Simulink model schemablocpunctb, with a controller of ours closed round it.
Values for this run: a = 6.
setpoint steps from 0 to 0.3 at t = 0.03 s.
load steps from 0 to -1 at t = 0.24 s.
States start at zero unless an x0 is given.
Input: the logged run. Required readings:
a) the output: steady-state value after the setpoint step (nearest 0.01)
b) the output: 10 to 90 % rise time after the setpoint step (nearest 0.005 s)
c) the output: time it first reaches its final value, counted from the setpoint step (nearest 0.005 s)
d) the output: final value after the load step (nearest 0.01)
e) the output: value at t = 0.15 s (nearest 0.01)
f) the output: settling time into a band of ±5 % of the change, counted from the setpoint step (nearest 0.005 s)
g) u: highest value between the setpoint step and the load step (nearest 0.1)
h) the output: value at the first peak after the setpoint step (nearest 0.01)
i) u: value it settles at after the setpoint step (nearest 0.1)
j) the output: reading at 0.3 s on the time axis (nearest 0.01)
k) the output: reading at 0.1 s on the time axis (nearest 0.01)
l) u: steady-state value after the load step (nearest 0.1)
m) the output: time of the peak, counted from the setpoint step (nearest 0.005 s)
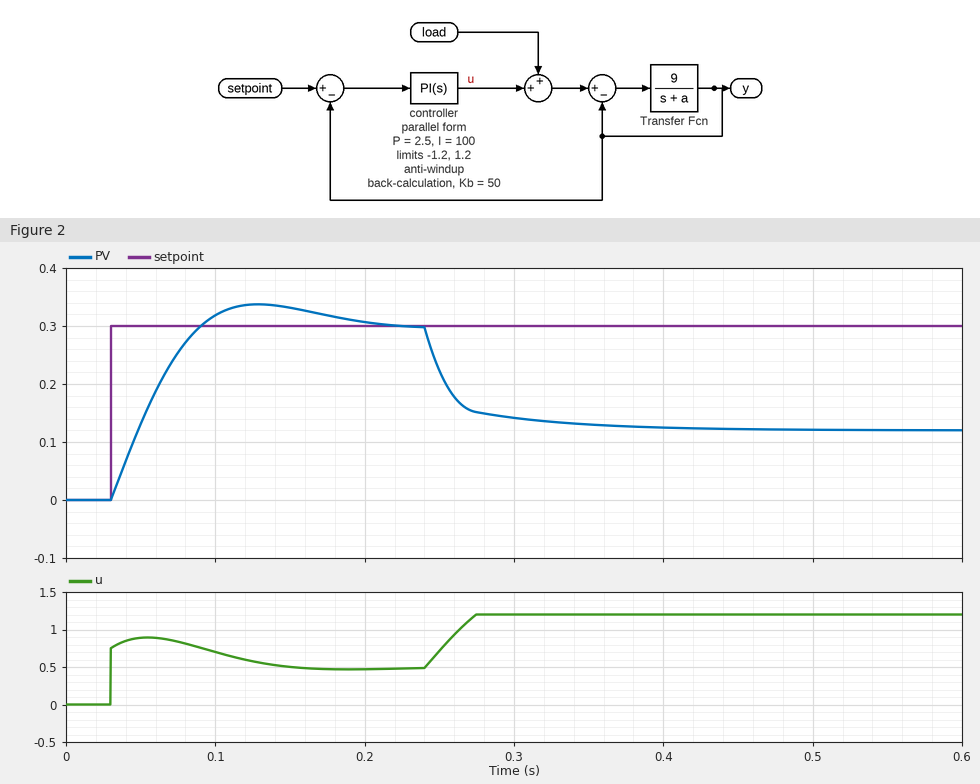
0.30
0.045 s
0.060 s
0.12
0.33
0.150 s
0.9
0.34
0.5
0.14
0.32
1.2
0.100 s
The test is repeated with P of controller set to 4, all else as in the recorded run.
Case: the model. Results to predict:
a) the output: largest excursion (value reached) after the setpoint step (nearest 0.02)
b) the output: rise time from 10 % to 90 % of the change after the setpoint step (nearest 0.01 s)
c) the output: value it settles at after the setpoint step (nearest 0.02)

0.32
0.04 s
0.30
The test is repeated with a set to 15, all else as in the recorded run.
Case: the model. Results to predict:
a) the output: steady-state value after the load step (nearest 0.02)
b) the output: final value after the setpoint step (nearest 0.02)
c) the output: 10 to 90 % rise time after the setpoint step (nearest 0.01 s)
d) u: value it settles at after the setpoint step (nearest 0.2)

0.08
0.30
0.06 s
0.8
